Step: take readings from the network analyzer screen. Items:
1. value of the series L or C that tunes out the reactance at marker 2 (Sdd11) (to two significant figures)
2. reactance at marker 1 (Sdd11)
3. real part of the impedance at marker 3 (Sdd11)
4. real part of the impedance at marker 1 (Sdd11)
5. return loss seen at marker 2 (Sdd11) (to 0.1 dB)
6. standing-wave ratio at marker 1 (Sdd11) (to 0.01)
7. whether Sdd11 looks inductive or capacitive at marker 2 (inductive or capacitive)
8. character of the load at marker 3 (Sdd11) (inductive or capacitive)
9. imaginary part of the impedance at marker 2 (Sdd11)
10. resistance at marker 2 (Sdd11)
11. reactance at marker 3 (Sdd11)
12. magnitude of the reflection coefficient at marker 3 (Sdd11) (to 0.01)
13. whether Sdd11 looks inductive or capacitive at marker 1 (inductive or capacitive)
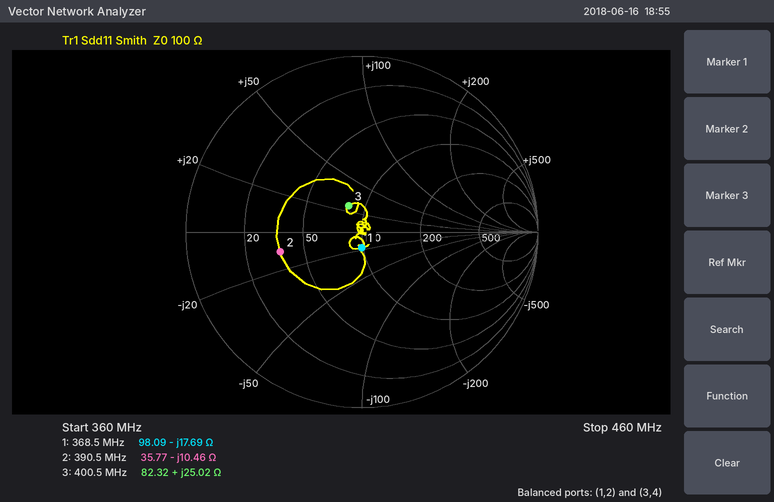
4.3 nH
-17.69 Ω
82.32 Ω
98.09 Ω
6.4 dB
1.20
capacitive
inductive
-10.46 Ω
35.77 Ω
+25.02 Ω
0.17
capacitive
